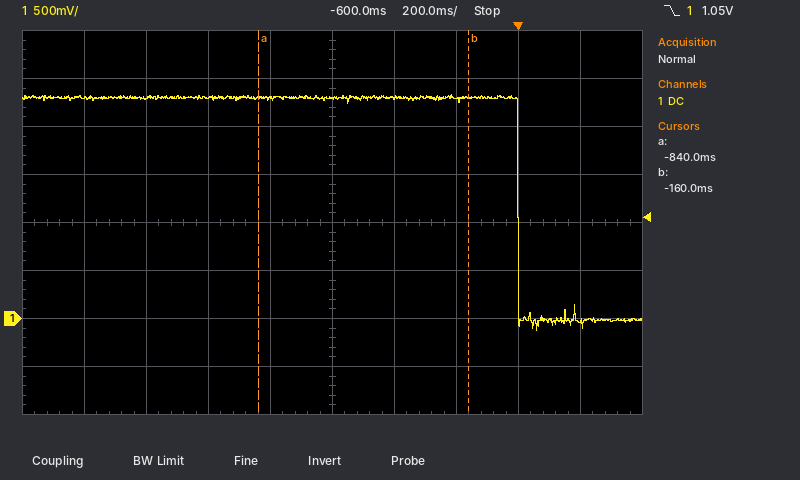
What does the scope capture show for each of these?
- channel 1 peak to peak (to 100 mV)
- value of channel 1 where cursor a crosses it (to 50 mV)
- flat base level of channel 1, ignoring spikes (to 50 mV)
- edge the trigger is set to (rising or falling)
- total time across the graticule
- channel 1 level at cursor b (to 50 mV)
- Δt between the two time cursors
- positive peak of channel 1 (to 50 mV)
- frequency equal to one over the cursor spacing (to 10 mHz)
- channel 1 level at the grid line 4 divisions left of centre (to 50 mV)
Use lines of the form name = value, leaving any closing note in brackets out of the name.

channel 1 peak to peak = 2.50 V
value of channel 1 where cursor a crosses it = 2.30 V
flat base level of channel 1, ignoring spikes = 0 mV
edge the trigger is set to = falling
total time across the graticule = 2 s
channel 1 level at cursor b = 2.30 V
Δt between the two time cursors = 680 ms
positive peak of channel 1 = 2.35 V
frequency equal to one over the cursor spacing = 1.47 Hz
channel 1 level at the grid line 4 divisions left of centre = 2.30 V
